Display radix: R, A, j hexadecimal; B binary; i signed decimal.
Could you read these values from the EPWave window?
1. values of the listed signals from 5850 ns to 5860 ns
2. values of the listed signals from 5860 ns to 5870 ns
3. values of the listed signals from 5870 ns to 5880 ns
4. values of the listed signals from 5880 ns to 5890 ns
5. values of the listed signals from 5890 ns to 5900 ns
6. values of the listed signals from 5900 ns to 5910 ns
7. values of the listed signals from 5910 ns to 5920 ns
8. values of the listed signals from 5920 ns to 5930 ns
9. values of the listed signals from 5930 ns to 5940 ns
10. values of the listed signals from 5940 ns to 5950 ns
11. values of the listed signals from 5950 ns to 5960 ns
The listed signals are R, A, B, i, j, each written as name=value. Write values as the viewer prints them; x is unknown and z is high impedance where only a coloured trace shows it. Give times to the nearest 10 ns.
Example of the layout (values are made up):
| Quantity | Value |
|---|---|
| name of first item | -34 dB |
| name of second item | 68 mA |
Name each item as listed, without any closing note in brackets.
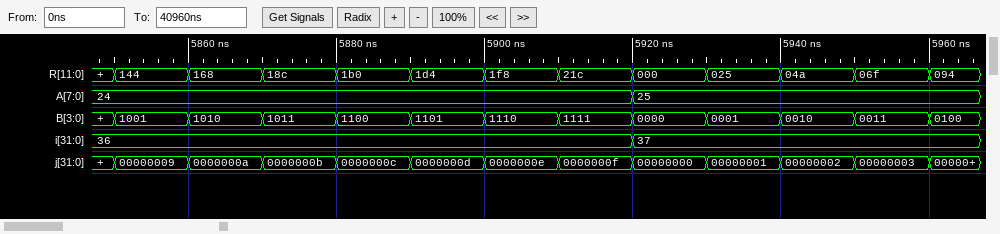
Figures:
| Quantity | Value |
|---|---|
| values of the listed signals from 5850 ns to 5860 ns | R=144, A=24, B=1001, i=36, j=00000009 |
| values of the listed signals from 5860 ns to 5870 ns | R=168, A=24, B=1010, i=36, j=0000000a |
| values of the listed signals from 5870 ns to 5880 ns | R=18c, A=24, B=1011, i=36, j=0000000b |
| values of the listed signals from 5880 ns to 5890 ns | R=1b0, A=24, B=1100, i=36, j=0000000c |
| values of the listed signals from 5890 ns to 5900 ns | R=1d4, A=24, B=1101, i=36, j=0000000d |
| values of the listed signals from 5900 ns to 5910 ns | R=1f8, A=24, B=1110, i=36, j=0000000e |
| values of the listed signals from 5910 ns to 5920 ns | R=21c, A=24, B=1111, i=36, j=0000000f |
| values of the listed signals from 5920 ns to 5930 ns | R=000, A=25, B=0000, i=37, j=00000000 |
| values of the listed signals from 5930 ns to 5940 ns | R=025, A=25, B=0001, i=37, j=00000001 |
| values of the listed signals from 5940 ns to 5950 ns | R=04a, A=25, B=0010, i=37, j=00000002 |
| values of the listed signals from 5950 ns to 5960 ns | R=06f, A=25, B=0011, i=37, j=00000003 |
